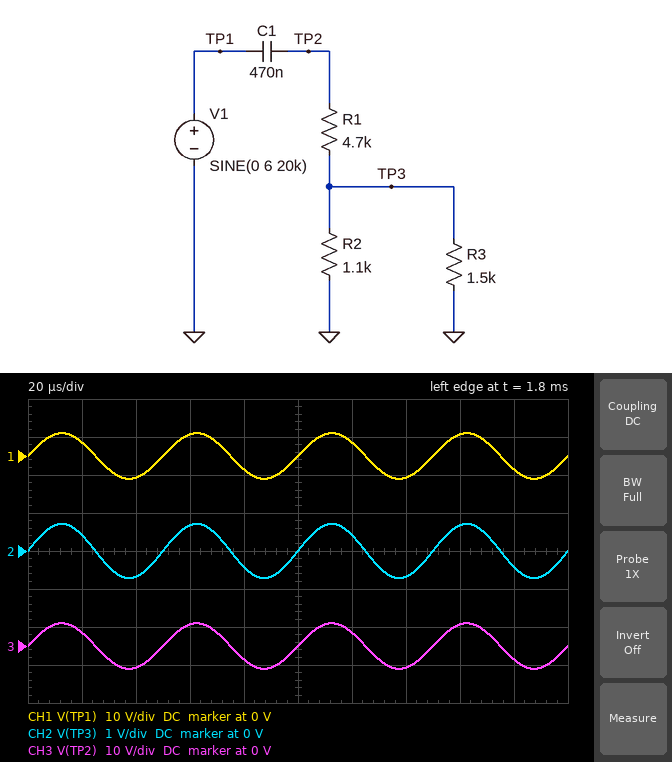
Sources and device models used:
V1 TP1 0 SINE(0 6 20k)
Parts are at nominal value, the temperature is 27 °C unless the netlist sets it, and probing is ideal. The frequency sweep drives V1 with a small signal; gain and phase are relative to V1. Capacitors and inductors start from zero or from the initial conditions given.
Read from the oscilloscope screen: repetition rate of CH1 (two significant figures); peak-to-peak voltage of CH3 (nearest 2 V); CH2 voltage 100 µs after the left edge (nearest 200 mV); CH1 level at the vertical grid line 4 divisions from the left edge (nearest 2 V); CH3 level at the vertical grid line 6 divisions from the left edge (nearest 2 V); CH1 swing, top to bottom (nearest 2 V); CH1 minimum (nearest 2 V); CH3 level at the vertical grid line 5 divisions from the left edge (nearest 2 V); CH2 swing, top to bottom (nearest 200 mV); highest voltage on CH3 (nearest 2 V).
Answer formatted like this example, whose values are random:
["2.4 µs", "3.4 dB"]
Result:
["20 kHz", "12 V", "0 V", "-4 V", "4 V", "12 V", "-6 V", "0 V", "1.4 V", "6 V"]
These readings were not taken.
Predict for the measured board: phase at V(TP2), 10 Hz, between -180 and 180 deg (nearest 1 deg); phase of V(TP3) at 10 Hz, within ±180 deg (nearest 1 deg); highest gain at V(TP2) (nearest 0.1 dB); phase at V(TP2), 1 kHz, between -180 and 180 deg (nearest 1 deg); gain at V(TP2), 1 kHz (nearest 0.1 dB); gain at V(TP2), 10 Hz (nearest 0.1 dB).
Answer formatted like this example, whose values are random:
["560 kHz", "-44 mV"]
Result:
["81 deg", "81 deg", "0 dB", "4 deg", "0 dB", "-16.2 dB"]
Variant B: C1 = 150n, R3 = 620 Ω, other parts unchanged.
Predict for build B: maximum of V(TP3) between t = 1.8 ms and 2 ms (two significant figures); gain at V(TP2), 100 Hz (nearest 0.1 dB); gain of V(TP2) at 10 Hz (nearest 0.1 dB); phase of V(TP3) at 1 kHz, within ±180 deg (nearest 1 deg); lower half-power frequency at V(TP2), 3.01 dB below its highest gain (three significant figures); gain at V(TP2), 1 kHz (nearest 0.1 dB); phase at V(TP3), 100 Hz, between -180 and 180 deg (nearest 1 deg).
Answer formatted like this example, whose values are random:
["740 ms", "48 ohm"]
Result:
["470 mV", "-7.3 dB", "-26.4 dB", "12 deg", "208 Hz", "-0.2 dB", "64 deg"]
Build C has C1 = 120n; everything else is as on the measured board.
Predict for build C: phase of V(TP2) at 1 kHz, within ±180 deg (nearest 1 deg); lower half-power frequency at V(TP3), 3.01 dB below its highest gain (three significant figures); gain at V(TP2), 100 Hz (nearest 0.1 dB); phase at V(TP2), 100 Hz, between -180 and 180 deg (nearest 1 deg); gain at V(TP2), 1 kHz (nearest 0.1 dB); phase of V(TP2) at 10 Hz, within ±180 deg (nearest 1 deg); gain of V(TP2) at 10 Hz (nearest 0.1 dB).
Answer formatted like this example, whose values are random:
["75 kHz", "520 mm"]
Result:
["14 deg", "249 Hz", "-8.6 dB", "68 deg", "-0.3 dB", "88 deg", "-27.9 dB"]
